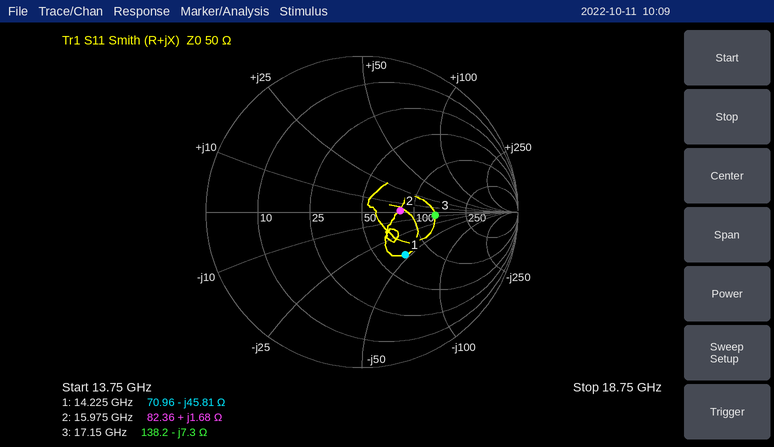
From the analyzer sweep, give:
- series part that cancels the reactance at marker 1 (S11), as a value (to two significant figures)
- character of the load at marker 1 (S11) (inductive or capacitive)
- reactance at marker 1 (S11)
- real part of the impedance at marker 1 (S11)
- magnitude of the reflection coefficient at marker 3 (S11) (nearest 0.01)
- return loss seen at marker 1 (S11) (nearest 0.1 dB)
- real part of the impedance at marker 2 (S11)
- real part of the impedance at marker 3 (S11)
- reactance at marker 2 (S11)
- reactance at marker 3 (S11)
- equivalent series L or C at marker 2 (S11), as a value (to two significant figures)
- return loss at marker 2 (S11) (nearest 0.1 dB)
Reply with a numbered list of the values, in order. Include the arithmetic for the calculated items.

1. L = 45.81 Ω/(2π × 14.225 GHz) ≈ 513 pH, so 510 pH to two significant figures
2. capacitive
3. -45.81 Ω
4. 70.96 Ω
5. 0.47
6. 8.2 dB
7. 82.36 Ω
8. 138.2 Ω
9. +1.68 Ω
10. -7.3 Ω
11. L = 1.68 Ω/(2π × 15.975 GHz) ≈ 17 pH
12. 12.2 dB
